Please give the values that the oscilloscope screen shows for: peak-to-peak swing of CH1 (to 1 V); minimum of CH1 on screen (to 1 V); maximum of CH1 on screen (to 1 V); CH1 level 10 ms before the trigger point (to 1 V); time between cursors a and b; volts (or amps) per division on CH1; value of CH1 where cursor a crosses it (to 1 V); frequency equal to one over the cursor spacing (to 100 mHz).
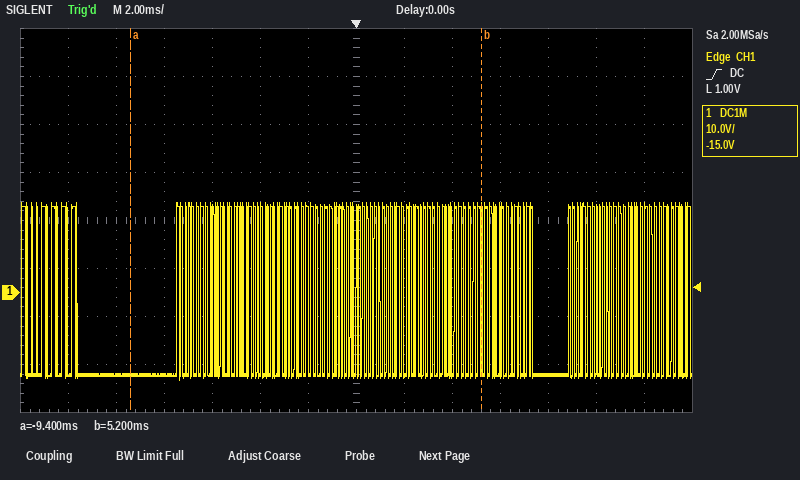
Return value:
37 V
-18 V
19 V
-17 V
14.6 ms
10 V
-17 V
68.5 Hz
